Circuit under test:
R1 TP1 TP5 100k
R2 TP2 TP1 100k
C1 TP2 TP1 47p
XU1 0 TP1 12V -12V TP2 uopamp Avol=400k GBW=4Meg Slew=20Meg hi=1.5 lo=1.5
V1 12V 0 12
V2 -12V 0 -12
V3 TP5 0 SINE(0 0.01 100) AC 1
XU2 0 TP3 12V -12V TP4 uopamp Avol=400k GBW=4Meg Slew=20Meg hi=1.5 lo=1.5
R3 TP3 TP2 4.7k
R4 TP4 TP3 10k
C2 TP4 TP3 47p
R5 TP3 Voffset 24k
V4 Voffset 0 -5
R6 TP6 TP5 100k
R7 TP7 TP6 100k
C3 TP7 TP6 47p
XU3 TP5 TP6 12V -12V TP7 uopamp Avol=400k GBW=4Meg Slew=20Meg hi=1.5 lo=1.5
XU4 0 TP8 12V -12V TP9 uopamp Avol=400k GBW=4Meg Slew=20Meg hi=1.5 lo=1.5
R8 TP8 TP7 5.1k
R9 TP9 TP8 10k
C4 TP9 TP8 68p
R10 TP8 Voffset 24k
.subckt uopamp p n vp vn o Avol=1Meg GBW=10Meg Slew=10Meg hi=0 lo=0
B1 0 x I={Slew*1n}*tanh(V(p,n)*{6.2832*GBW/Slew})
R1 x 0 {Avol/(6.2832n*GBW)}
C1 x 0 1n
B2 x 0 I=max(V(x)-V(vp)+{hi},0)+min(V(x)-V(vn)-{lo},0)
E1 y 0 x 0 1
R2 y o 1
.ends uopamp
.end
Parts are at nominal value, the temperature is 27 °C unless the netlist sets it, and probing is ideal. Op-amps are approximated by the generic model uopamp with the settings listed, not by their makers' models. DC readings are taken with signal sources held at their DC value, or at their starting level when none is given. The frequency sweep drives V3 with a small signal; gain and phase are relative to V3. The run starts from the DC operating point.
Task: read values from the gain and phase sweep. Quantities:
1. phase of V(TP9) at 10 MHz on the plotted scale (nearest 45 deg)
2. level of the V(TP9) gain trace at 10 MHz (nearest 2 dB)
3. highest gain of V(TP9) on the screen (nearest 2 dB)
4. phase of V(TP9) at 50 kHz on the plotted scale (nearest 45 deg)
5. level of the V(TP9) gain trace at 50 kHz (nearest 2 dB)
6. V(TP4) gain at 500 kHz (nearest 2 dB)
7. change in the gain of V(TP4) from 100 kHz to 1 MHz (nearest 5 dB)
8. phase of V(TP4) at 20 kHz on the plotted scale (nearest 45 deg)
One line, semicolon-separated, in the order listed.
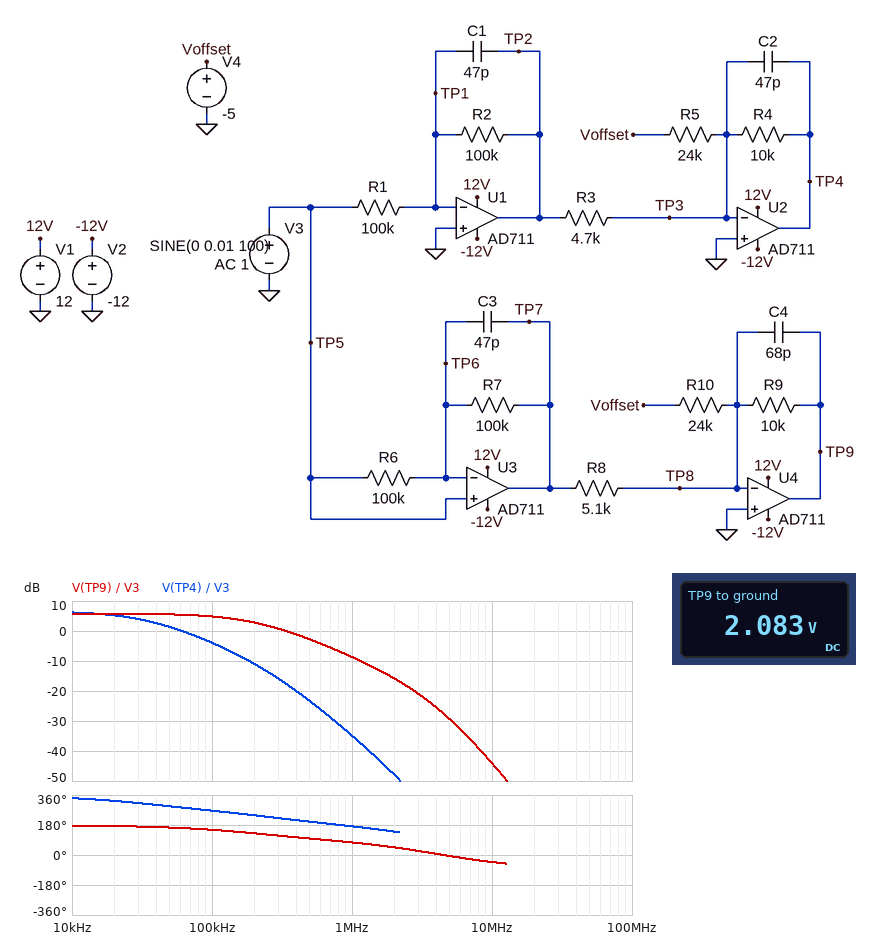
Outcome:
-45 deg; -44 dB; 6 dB; 180 deg; 6 dB; -24 dB; -30 dB; 315 deg
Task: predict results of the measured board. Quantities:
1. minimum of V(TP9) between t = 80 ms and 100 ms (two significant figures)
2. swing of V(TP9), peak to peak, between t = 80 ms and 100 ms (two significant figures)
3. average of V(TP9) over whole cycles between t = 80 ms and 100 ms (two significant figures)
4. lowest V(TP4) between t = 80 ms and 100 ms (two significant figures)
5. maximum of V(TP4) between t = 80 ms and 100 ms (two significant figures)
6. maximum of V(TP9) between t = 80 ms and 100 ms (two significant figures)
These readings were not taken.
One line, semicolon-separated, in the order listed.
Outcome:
2.1 V; 39 mV; 2.1 V; 2.1 V; 2.1 V; 2.1 V
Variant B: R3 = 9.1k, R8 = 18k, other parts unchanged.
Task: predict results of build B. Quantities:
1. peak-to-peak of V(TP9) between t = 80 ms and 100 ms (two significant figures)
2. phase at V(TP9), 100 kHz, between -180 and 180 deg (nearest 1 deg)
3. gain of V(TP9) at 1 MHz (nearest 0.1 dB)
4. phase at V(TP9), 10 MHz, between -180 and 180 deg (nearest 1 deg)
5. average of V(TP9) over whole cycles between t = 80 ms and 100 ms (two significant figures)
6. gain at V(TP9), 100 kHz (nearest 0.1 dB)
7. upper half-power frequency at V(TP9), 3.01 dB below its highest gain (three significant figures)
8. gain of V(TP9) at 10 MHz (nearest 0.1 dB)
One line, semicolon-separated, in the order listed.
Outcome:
11 mV; 153 deg; -19.0 dB; -44 deg; 2.1 V; -6.0 dB; 216 kHz; -54.9 dB
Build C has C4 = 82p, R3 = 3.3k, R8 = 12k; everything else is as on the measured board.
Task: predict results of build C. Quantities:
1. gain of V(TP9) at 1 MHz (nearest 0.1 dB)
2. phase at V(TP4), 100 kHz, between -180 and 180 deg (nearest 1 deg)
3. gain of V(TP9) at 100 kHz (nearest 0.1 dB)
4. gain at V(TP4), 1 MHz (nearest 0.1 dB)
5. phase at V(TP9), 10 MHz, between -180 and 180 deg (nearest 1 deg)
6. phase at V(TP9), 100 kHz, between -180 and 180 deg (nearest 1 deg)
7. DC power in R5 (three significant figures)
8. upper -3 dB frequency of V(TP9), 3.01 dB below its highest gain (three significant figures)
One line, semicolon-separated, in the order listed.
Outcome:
-17.1 dB; -95 deg; -2.8 dB; -32.3 dB; -44 deg; 148 deg; 1.04 mW; 179 kHz
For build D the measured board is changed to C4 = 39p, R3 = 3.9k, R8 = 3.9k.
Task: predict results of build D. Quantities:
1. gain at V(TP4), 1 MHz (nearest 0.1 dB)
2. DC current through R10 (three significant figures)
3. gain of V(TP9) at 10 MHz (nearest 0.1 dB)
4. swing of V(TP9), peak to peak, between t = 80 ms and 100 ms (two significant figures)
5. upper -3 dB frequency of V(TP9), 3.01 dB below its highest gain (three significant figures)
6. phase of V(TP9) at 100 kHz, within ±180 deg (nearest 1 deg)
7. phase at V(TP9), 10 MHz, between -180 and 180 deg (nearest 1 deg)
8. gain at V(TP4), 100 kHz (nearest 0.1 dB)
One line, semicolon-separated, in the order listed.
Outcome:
-33.5 dB; 208 µA; -37.2 dB; 51 mV; 299 kHz; 159 deg; -38 deg; -2.3 dB
